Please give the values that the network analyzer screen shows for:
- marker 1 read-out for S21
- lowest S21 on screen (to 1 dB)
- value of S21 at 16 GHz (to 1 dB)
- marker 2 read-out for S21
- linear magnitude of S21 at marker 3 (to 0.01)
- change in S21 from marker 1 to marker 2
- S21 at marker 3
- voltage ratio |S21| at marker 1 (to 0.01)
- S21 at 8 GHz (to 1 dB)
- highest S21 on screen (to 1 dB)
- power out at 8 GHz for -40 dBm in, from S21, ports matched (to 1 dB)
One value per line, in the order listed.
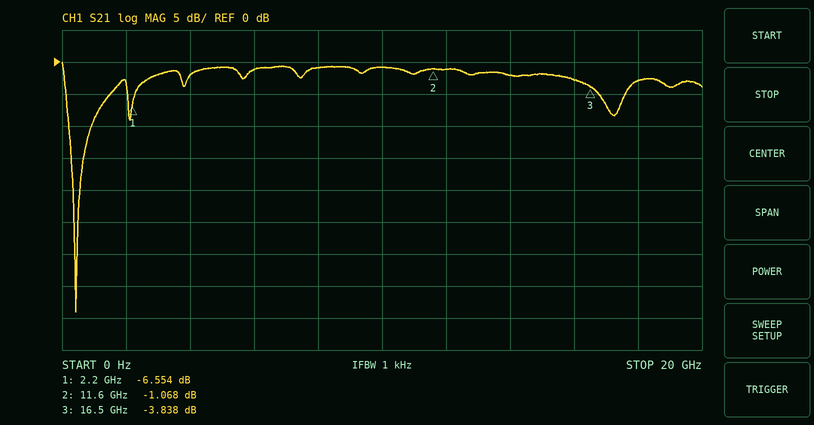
-6.554 dB
-39 dB
-3 dB
-1.068 dB
0.64
5.486 dB
-3.838 dB
0.47
-1 dB
0 dB
-41 dBm
